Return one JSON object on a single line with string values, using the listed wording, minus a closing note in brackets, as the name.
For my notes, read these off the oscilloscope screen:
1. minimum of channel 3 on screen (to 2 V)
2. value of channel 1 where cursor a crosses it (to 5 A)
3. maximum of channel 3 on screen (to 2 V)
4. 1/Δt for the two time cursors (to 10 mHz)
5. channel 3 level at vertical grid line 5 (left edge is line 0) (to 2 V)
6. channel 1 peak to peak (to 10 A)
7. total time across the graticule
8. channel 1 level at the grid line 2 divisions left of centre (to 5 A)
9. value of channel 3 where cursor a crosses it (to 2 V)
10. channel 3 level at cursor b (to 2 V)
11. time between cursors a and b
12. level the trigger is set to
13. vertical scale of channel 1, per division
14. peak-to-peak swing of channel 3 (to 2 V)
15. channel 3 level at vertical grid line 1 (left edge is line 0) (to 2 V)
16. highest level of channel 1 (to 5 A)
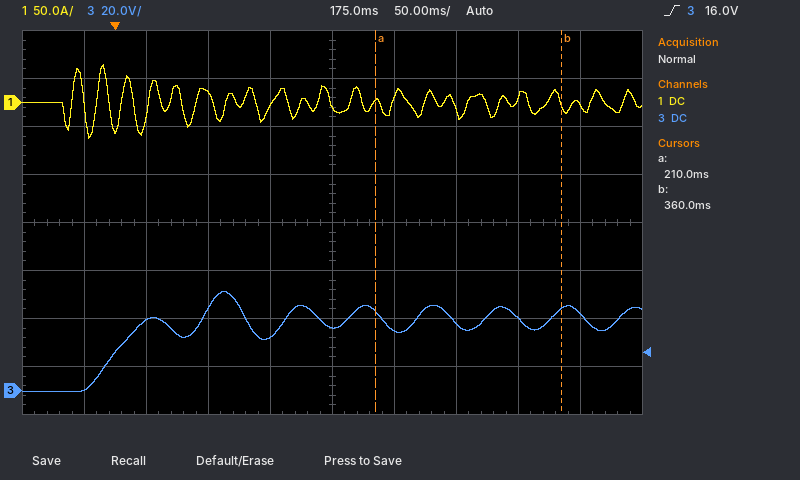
{"minimum of channel 3 on screen": "0 V", "value of channel 1 where cursor a crosses it": "0 A", "maximum of channel 3 on screen": "42 V", "1/Δt for the two time cursors": "6.67 Hz", "channel 3 level at vertical grid line 5 (left edge is line 0)": "26 V", "channel 1 peak to peak": "80 A", "total time across the graticule": "500 ms", "channel 1 level at the grid line 2 divisions left of centre": "10 A", "value of channel 3 where cursor a crosses it": "32 V", "channel 3 level at cursor b": "34 V", "time between cursors a and b": "150 ms", "level the trigger is set to": "16.0 V", "vertical scale of channel 1, per division": "50 A", "peak-to-peak swing of channel 3": "42 V", "channel 3 level at vertical grid line 1 (left edge is line 0)": "0 V", "highest level of channel 1": "40 A"}
